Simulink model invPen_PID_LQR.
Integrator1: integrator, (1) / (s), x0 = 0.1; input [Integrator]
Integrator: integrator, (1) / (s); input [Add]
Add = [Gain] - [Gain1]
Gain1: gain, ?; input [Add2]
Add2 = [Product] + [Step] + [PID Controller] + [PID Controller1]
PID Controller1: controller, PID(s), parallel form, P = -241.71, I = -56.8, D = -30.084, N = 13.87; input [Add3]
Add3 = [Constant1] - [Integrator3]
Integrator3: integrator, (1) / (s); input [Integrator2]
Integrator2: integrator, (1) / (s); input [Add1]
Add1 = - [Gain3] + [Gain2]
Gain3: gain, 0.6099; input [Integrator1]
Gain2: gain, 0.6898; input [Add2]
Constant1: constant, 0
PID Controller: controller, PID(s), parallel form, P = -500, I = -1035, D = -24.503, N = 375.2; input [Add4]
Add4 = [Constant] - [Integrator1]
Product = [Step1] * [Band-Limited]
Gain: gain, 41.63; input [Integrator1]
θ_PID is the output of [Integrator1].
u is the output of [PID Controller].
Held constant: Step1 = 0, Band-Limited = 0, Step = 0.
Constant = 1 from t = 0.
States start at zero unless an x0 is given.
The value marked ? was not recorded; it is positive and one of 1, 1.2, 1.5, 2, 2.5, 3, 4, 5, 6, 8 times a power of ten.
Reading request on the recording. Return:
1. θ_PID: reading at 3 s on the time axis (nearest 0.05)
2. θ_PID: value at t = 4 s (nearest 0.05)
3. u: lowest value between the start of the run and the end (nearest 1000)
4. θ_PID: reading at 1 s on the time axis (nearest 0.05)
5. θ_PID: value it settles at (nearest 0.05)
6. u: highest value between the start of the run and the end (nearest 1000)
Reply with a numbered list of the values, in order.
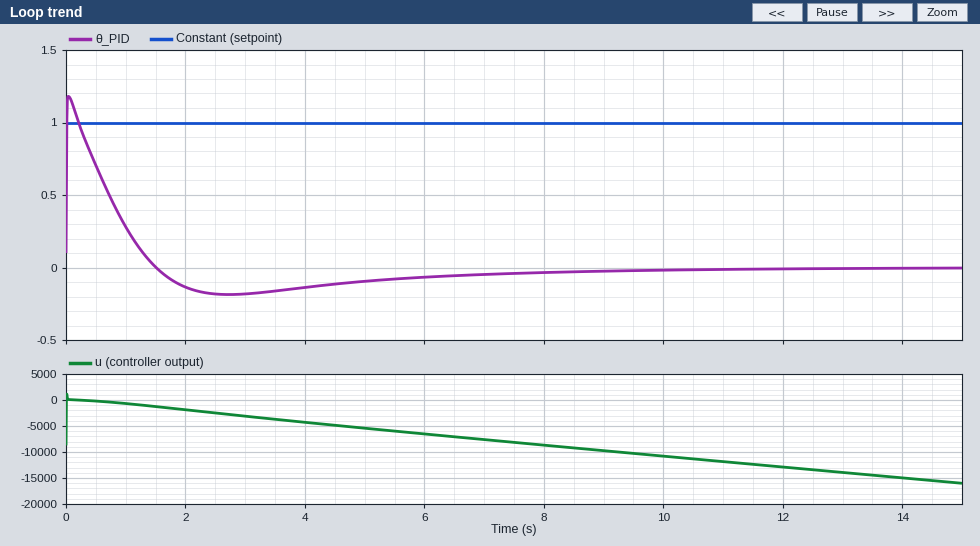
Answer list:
1. -0.20
2. -0.15
3. -16000
4. 0.30
5. 0.00
6. 1000
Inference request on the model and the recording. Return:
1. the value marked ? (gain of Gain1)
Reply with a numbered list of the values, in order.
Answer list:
1. 5
